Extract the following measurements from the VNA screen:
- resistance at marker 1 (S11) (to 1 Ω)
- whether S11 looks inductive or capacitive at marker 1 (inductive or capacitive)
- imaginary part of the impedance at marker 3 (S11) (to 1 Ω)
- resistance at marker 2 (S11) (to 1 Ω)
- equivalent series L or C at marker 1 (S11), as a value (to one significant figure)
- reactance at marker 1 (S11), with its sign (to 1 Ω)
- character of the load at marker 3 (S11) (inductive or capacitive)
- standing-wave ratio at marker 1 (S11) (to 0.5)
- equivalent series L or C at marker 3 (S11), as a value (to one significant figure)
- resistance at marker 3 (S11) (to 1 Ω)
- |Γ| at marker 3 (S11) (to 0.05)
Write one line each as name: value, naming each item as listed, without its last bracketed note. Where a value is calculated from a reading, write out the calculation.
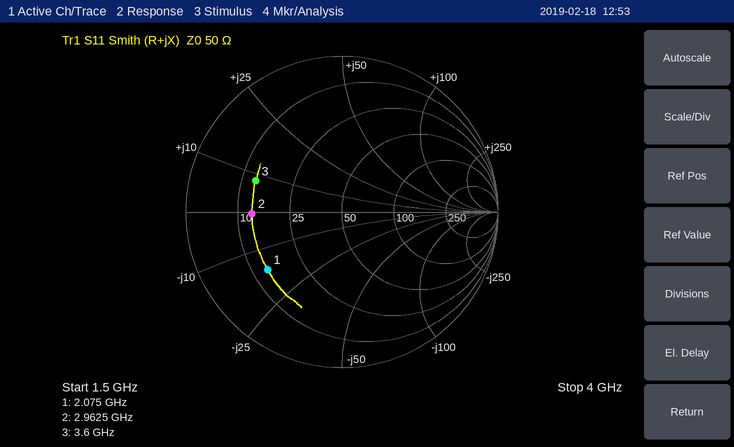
resistance at marker 1 (S11): 14 Ω
whether S11 looks inductive or capacitive at marker 1: capacitive
imaginary part of the impedance at marker 3 (S11): +8 Ω
resistance at marker 2 (S11): 13 Ω
equivalent series L or C at marker 1 (S11), as a value: C = 1/(2π × 2.075 GHz × 16 Ω) ≈ 5 pF
reactance at marker 1 (S11), with its sign: -16 Ω
character of the load at marker 3 (S11): inductive
standing-wave ratio at marker 1 (S11): 4.0
equivalent series L or C at marker 3 (S11), as a value: L = 8 Ω/(2π × 3.6 GHz) ≈ 354 pH, so 400 pH to one significant figure
resistance at marker 3 (S11): 13 Ω
|Γ| at marker 3 (S11): 0.60
